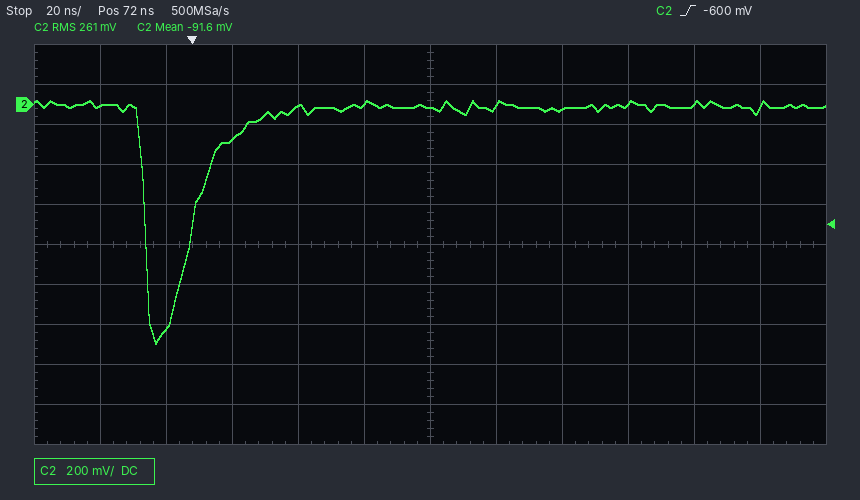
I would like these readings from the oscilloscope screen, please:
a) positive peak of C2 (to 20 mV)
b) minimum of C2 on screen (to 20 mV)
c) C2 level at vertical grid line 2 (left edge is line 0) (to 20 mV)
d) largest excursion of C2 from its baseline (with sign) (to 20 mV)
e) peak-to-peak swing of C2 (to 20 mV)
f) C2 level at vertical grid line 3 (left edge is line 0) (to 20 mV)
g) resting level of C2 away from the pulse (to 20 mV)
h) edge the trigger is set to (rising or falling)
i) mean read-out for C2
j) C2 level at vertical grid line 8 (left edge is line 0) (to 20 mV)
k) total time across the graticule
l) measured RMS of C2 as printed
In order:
20 mV
-1.20 V
-1.12 V
-1.18 V
1.22 V
-180 mV
-20 mV
rising
-91.6 mV
-20 mV
240 ns
261 mV
